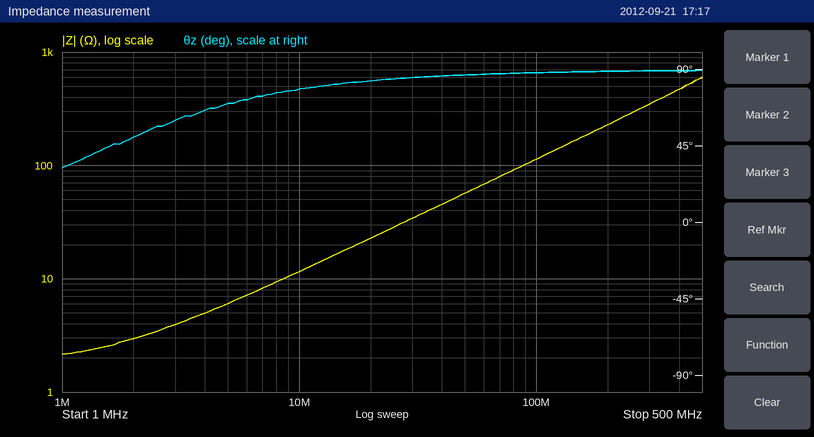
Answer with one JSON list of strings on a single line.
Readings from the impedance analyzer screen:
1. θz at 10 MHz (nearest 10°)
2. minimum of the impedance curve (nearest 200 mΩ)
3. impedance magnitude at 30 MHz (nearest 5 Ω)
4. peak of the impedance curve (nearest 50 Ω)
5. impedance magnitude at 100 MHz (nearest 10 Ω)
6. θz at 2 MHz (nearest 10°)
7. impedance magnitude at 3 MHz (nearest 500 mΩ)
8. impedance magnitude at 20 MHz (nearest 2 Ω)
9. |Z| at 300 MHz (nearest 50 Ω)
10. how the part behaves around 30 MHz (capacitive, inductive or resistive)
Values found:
["80°", "2.2 Ω", "35 Ω", "600 Ω", "110 Ω", "50°", "4.0 Ω", "22 Ω", "350 Ω", "inductive"]
